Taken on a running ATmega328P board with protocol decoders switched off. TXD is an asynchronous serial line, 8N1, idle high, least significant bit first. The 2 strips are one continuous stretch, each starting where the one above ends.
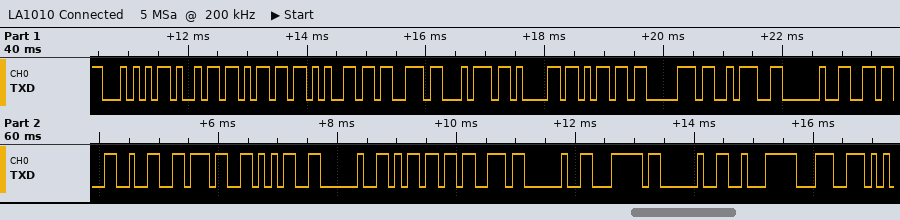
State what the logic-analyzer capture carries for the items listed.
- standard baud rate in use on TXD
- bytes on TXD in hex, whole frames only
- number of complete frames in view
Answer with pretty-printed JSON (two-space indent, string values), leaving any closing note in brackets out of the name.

{
  "standard baud rate in use on TXD": "9600 baud",
  "bytes on TXD in hex, whole frames only": "54 69 6D 65 73 74 61 6D 70 3A 20 36 32 37 35 20 6D 73 20 7C 20 E2 9C",
  "number of complete frames in view": "23"
}
